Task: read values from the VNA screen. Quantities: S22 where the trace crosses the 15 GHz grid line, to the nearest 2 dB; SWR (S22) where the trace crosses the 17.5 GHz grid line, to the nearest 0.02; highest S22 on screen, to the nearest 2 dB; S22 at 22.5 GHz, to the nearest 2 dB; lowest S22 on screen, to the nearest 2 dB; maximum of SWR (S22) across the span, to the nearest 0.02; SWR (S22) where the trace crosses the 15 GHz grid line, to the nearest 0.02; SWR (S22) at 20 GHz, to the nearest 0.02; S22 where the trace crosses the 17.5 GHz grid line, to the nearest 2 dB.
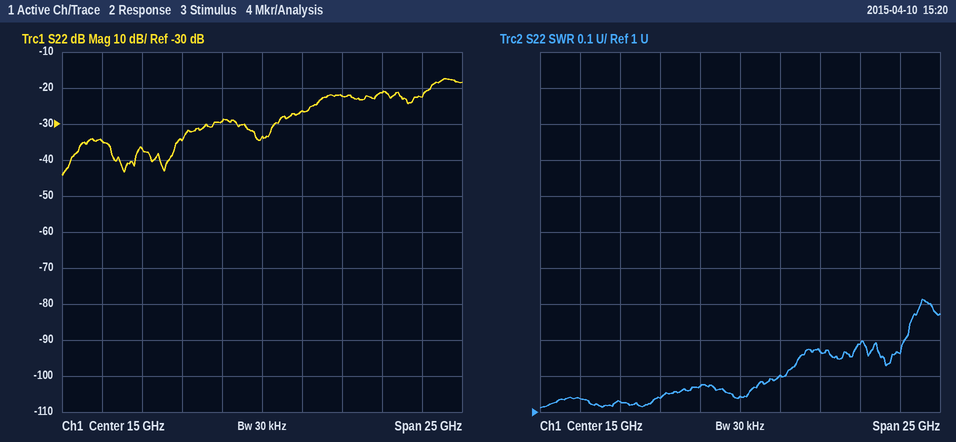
-34 dB
1.10
-18 dB
-22 dB
-44 dB
1.32
1.04
1.16
-26 dB
